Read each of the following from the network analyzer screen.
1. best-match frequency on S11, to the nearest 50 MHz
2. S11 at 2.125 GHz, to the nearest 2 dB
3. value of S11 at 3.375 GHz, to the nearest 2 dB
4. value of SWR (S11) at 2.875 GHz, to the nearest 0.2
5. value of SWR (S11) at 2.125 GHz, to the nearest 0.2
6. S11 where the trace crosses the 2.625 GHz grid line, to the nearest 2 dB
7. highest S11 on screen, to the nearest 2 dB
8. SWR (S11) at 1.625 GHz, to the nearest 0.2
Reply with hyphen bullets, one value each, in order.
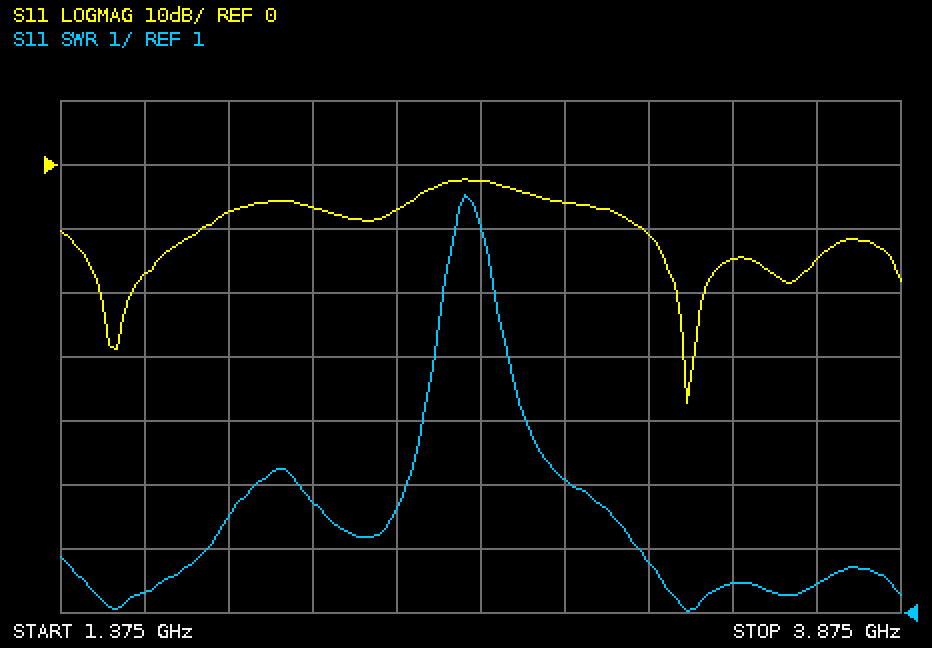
- 3.25 GHz
- -6 dB
- -14 dB
- 3.0
- 2.8
- -2 dB
- -2 dB
- 1.4
